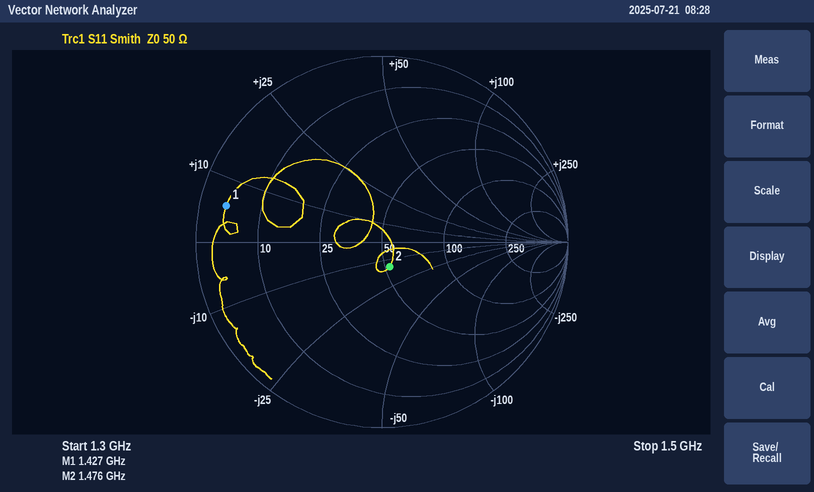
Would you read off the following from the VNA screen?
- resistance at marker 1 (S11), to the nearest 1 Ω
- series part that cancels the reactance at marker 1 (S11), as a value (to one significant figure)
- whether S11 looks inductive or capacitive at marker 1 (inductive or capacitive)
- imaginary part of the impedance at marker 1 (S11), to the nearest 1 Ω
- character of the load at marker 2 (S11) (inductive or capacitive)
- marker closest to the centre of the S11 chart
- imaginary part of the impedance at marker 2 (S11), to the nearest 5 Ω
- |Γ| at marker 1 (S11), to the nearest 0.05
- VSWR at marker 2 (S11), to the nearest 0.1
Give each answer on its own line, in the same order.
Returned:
4 Ω
20 pF
inductive
+6 Ω
capacitive
marker 2
-15 Ω
0.85
1.3
